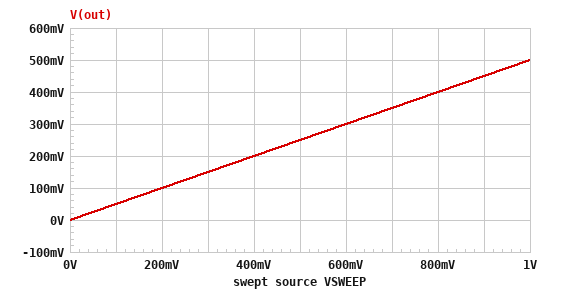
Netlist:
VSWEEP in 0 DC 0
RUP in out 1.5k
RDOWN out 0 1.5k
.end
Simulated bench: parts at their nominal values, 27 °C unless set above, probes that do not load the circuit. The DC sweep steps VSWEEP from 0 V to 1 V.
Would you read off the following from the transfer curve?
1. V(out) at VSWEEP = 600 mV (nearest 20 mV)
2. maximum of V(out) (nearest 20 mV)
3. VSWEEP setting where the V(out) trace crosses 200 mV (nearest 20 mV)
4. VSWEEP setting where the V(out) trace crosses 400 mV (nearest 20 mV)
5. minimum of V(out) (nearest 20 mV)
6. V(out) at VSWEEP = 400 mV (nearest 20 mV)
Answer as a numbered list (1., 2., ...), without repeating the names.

1. 300 mV
2. 500 mV
3. 400 mV
4. 800 mV
5. 0 V
6. 200 mV
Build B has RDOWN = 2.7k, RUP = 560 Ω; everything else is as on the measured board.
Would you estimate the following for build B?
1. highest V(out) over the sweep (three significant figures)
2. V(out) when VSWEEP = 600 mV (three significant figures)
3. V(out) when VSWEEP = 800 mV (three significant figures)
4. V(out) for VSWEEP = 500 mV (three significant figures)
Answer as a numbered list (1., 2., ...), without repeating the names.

1. 828 mV
2. 497 mV
3. 663 mV
4. 414 mV
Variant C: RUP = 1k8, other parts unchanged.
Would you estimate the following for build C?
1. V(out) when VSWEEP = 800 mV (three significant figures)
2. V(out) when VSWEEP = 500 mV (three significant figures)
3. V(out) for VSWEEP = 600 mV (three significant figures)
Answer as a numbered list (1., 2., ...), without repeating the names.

1. 364 mV
2. 227 mV
3. 273 mV
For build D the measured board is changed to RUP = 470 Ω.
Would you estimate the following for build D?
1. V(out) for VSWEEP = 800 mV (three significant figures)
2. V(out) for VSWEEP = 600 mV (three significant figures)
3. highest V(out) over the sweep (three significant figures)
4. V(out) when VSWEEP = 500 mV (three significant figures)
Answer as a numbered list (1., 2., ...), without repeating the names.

1. 609 mV
2. 457 mV
3. 761 mV
4. 381 mV
